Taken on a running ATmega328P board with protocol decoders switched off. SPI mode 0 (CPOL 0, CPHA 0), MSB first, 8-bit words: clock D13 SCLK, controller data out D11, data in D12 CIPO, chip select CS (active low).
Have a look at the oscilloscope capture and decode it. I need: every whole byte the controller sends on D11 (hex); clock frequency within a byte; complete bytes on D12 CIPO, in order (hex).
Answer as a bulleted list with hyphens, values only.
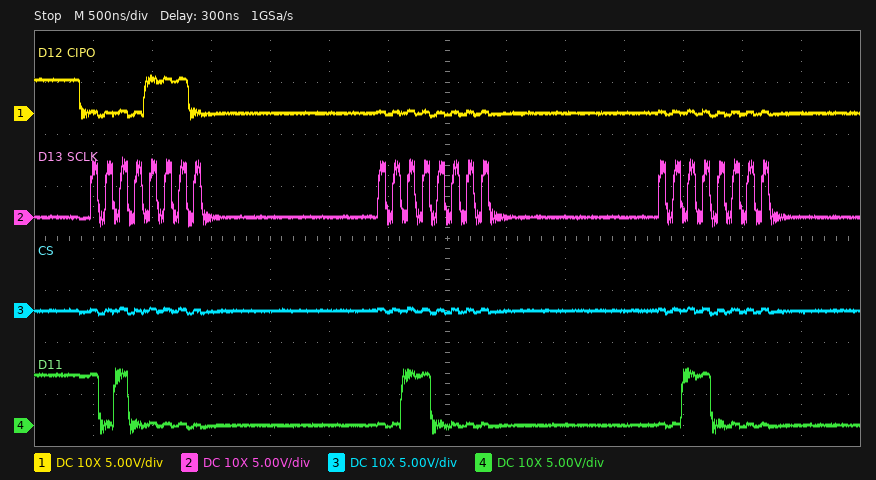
- 0xA0 0x30 0x30
- 8 MHz
- 0x0E 0x00 0x00
